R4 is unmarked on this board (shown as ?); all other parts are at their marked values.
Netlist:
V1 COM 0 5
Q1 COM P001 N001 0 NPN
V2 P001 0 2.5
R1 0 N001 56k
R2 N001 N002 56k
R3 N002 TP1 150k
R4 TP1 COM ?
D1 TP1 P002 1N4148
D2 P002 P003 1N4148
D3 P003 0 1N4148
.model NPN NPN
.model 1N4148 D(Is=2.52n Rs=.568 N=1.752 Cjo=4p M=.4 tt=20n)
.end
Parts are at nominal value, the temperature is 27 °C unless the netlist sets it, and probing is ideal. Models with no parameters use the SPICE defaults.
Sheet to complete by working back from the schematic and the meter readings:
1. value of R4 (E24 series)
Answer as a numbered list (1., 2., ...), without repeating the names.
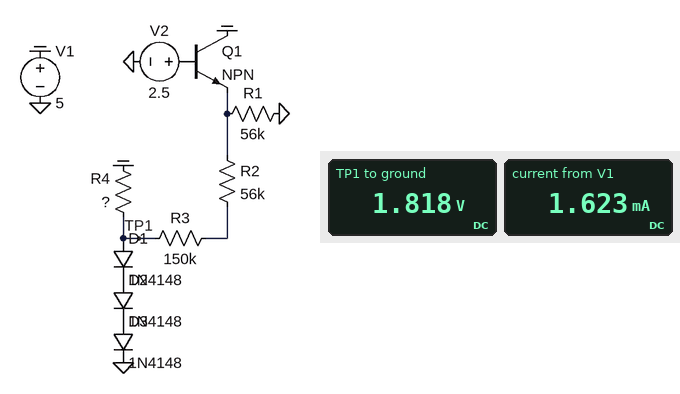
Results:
1. 2 kΩ
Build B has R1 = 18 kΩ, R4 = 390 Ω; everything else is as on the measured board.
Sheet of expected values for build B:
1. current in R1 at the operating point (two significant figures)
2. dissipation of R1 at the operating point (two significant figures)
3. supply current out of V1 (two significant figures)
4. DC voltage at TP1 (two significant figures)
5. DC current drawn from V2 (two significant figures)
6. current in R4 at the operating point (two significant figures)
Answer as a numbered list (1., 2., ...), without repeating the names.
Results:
1. 99 µA
2. 180 µW
3. 7.7 mA
4. 2.0 V
5. 970 nA
6. 7.6 mA
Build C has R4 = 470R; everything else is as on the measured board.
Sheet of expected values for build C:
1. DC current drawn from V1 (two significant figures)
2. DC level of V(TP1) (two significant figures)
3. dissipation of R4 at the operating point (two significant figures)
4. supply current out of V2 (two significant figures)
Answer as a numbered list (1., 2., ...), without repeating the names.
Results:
1. 6.4 mA
2. 2.0 V
3. 19 mW
4. 310 nA
